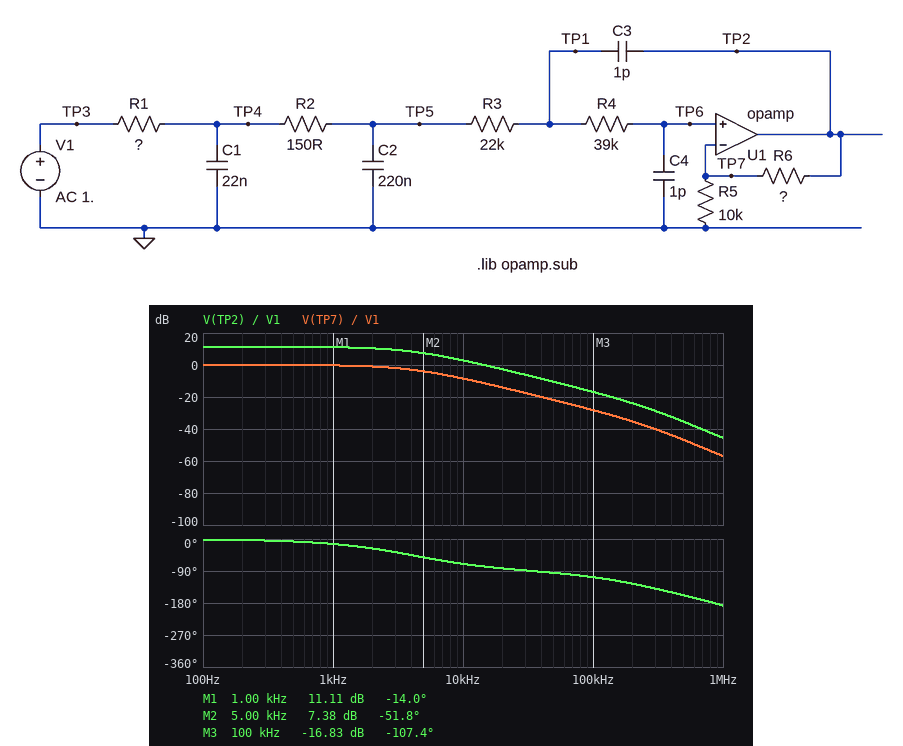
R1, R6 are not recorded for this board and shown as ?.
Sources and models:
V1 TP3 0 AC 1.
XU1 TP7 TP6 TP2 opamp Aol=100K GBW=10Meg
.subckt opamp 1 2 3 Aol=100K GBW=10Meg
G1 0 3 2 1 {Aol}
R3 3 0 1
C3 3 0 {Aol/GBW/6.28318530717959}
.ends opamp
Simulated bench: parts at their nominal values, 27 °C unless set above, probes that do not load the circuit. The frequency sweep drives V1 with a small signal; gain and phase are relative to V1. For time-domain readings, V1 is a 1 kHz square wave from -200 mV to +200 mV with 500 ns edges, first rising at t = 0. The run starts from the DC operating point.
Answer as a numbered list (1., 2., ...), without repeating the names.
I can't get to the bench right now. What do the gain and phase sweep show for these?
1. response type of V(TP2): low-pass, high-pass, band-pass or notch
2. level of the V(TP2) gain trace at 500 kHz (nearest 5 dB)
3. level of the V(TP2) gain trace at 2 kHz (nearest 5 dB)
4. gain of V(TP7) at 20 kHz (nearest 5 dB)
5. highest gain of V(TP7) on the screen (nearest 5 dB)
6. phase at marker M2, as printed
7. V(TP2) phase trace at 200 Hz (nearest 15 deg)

1. low-pass
2. -35 dB
3. 10 dB
4. -15 dB
5. 0 dB
6. -51.8 deg
7. 0 deg
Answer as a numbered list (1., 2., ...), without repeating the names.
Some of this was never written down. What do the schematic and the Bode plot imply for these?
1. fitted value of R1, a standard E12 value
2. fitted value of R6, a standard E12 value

1. 27 Ω
2. 27 kΩ
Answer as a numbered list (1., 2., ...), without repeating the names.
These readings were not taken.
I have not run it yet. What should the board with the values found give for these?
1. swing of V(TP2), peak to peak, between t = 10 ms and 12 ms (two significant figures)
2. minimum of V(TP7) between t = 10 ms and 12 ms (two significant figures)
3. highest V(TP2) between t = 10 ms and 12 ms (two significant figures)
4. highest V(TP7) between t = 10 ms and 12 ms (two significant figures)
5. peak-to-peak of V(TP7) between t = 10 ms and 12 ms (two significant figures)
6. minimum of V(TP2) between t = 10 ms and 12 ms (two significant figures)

1. 1.5 V
2. -200 mV
3. 740 mV
4. 200 mV
5. 400 mV
6. -740 mV
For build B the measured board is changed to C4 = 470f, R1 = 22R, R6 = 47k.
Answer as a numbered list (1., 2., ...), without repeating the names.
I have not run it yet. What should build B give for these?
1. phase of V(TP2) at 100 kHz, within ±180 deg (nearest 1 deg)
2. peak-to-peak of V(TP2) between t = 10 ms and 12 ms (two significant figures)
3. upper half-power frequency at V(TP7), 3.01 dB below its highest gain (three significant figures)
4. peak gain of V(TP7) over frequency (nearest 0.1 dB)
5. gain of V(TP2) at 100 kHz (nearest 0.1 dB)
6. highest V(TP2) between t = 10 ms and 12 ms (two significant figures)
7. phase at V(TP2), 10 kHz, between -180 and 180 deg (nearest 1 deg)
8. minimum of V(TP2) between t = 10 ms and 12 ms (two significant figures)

1. -103 deg
2. 2.3 V
3. 4.20 kHz
4. 0 dB
5. -12.7 dB
6. 1.1 V
7. -69 deg
8. -1.1 V
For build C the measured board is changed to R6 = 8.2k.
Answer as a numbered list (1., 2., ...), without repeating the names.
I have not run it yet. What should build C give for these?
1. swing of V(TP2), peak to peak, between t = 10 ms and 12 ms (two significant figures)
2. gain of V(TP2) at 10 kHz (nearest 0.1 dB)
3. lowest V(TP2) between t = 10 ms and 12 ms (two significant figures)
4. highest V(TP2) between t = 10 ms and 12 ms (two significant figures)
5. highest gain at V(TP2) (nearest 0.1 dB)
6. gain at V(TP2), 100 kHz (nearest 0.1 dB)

1. 730 mV
2. -3.3 dB
3. -360 mV
4. 360 mV
5. 5.2 dB
6. -23.0 dB
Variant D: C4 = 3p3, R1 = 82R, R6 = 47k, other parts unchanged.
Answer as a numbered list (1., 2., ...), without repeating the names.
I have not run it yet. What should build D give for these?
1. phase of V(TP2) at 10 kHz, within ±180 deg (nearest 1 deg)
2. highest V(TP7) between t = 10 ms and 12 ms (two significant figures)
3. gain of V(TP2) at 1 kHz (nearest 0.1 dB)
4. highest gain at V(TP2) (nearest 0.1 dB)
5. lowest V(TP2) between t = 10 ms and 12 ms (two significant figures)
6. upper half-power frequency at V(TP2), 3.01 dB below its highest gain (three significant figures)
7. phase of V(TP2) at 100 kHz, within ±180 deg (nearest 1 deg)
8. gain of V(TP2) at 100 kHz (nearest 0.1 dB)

1. -78 deg
2. 200 mV
3. 14.7 dB
4. 15.1 dB
5. -1.1 V
6. 3.08 kHz
7. -131 deg
8. -16.9 dB
